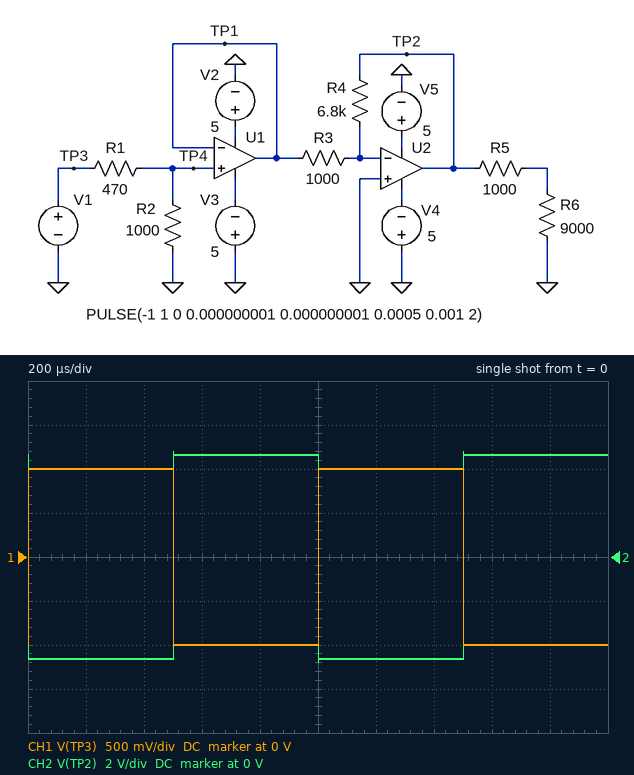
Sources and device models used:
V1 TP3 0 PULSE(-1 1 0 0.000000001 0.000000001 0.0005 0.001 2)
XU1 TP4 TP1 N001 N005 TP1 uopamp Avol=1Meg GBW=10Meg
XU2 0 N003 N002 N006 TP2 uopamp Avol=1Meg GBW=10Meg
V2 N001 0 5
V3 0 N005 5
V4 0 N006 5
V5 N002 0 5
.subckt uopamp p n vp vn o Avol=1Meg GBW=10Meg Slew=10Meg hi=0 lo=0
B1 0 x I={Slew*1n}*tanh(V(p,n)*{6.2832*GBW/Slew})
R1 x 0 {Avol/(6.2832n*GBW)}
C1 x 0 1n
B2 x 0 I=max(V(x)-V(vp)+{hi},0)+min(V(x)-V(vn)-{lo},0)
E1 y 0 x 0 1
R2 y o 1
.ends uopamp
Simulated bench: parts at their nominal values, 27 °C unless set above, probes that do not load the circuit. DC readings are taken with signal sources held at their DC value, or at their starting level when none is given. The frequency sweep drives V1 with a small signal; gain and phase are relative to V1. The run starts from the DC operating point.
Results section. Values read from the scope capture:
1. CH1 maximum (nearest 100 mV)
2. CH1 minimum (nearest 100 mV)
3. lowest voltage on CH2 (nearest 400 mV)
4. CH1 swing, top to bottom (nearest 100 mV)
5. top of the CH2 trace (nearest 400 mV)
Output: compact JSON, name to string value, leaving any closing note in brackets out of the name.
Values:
{"CH1 maximum": "1.0 V", "CH1 minimum": "-1.0 V", "lowest voltage on CH2": "-4.8 V", "CH1 swing, top to bottom": "2.0 V", "top of the CH2 trace": "4.8 V"}
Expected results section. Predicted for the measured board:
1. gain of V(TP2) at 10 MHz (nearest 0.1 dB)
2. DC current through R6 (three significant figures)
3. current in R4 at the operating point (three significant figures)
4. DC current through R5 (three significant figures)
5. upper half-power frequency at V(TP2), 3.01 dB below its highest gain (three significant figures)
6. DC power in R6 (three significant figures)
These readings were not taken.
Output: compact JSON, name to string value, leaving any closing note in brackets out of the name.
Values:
{"gain of V(TP2) at 10 MHz": "-7.6 dB", "DC current through R6": "463 µA", "current in R4 at the operating point": "680 µA", "DC current through R5": "463 µA", "upper half-power frequency at V(TP2), 3.01 dB below its highest gain": "1.26 MHz", "DC power in R6": "1.93 mW"}
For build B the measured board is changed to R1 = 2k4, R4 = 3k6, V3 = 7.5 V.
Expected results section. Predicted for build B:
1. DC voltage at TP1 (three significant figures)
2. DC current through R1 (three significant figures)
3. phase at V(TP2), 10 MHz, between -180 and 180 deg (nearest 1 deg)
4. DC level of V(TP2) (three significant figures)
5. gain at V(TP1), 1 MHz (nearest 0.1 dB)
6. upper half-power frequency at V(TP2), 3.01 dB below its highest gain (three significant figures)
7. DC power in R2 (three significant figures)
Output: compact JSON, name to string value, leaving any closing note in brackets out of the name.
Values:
{"DC voltage at TP1": "-294 mV", "DC current through R1": "294 µA", "phase at V(TP2), 10 MHz, between -180 and 180 deg": "57 deg", "DC level of V(TP2)": "1.06 V", "gain at V(TP1), 1 MHz": "-10.7 dB", "upper half-power frequency at V(TP2), 3.01 dB below its highest gain": "2.08 MHz", "DC power in R2": "86.5 µW"}
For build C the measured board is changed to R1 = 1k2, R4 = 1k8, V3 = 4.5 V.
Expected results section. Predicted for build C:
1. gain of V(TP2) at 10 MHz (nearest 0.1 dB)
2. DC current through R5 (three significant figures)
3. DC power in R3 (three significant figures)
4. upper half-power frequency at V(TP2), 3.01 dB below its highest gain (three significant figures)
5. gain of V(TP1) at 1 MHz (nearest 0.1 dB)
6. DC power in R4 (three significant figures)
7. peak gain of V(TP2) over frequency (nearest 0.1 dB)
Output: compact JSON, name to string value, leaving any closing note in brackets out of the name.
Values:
{"gain of V(TP2) at 10 MHz": "-14.2 dB", "DC current through R5": "81.8 µA", "DC power in R3": "207 µW", "upper half-power frequency at V(TP2), 3.01 dB below its highest gain": "3.22 MHz", "gain of V(TP1) at 1 MHz": "-6.9 dB", "DC power in R4": "372 µW", "peak gain of V(TP2) over frequency": "-1.7 dB"}
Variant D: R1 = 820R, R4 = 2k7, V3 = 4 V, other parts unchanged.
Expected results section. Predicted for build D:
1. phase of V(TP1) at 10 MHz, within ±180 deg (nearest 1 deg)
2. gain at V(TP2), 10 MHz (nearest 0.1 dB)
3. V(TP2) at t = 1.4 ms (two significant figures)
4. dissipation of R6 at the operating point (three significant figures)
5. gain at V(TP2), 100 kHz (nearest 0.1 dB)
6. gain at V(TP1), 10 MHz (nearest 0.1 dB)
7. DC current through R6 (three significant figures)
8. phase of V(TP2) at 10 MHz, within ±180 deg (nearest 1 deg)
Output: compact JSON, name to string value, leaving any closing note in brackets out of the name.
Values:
{"phase of V(TP1) at 10 MHz, within ±180 deg": "-45 deg", "gain at V(TP2), 10 MHz": "-11.3 dB", "V(TP2) at t = 1.4 ms": "-1.5 V", "dissipation of R6 at the operating point": "198 µW", "gain at V(TP2), 100 kHz": "3.4 dB", "gain at V(TP1), 10 MHz": "-8.2 dB", "DC current through R6": "148 µA", "phase of V(TP2) at 10 MHz, within ±180 deg": "60 deg"}
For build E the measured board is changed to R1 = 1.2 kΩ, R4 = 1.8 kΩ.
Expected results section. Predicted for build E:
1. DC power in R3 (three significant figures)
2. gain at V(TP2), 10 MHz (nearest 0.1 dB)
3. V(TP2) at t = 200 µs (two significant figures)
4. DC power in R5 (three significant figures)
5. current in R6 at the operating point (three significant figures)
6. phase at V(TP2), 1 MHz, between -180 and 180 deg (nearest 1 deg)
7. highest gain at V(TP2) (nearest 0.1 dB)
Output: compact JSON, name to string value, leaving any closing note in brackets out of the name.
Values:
{"DC power in R3": "207 µW", "gain at V(TP2), 10 MHz": "-14.2 dB", "V(TP2) at t = 200 µs": "-820 mV", "DC power in R5": "6.69 µW", "current in R6 at the operating point": "81.8 µA", "phase at V(TP2), 1 MHz, between -180 and 180 deg": "159 deg", "highest gain at V(TP2)": "-1.7 dB"}
